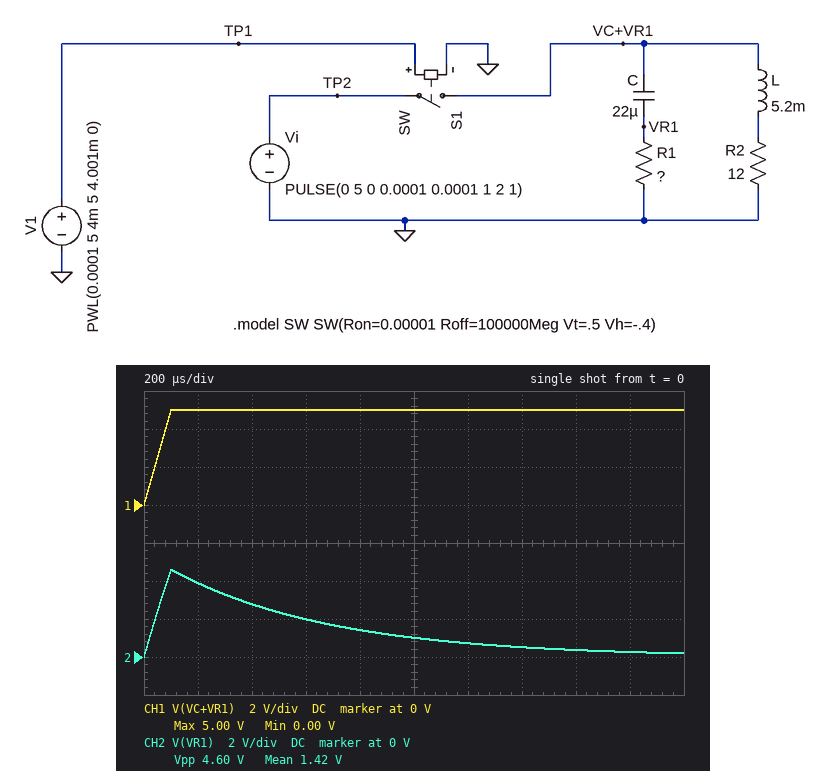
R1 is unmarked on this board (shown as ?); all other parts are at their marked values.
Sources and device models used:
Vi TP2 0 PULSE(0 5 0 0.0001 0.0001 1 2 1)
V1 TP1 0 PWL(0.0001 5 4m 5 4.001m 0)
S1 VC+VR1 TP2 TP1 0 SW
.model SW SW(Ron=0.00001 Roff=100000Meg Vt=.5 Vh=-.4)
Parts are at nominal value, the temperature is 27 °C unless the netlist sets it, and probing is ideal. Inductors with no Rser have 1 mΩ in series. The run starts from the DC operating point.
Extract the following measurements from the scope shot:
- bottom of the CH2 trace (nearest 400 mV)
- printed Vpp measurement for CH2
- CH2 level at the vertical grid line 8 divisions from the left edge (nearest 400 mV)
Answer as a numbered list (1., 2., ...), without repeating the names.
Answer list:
1. 0 V
2. 4.60 V
3. 400 mV
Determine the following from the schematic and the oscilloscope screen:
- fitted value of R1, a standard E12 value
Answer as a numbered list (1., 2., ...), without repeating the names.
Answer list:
1. 27 Ω
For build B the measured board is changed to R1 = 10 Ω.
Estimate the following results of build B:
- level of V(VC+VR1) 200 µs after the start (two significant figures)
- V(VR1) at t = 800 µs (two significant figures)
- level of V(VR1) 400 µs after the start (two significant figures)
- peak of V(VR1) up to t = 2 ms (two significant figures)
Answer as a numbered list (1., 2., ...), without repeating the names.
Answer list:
1. 5.0 V
2. 170 mV
3. 1.0 V
4. 4.0 V
